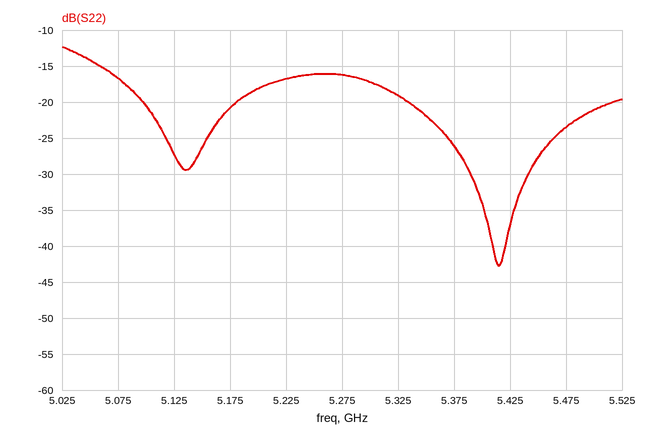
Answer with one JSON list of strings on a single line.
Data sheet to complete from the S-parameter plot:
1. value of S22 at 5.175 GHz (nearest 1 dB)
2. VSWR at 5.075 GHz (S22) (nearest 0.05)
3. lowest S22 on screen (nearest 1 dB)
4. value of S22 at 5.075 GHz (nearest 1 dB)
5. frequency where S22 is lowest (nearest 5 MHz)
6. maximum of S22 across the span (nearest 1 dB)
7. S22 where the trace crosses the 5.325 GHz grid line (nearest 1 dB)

["-21 dB", "1.35", "-43 dB", "-17 dB", "5.415 GHz", "-12 dB", "-19 dB"]
